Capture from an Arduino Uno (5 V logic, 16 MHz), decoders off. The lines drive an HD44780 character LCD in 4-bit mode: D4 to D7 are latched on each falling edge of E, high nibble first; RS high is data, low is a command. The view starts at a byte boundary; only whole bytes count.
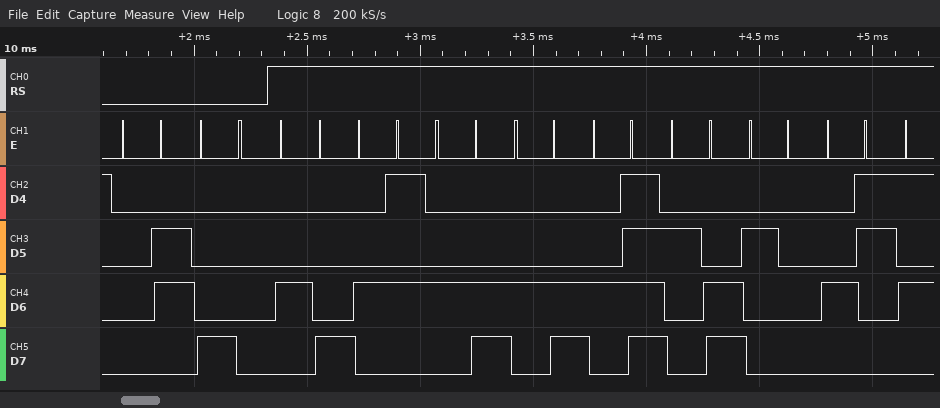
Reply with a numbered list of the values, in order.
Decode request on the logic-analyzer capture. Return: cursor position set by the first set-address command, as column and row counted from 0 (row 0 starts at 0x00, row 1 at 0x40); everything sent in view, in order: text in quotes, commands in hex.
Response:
1. column 0, row 0
2. 0x06 0x80 "HELLO, C"
